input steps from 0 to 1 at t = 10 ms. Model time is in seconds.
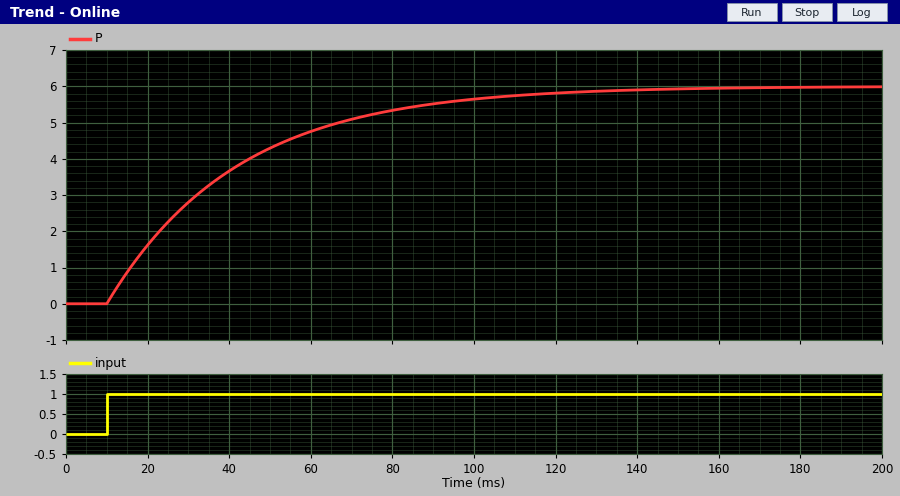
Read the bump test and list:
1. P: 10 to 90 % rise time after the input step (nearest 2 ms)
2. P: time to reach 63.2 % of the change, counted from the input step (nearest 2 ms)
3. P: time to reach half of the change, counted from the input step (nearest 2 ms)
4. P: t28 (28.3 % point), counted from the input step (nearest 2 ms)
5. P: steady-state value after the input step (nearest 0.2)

70 ms
32 ms
22 ms
10 ms
6.0
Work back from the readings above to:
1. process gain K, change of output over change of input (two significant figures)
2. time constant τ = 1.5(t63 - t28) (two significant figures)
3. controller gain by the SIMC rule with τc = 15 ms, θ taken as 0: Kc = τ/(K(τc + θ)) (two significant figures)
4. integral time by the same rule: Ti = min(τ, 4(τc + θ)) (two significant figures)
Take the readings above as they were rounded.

6.0
33 ms
0.37
33 ms
